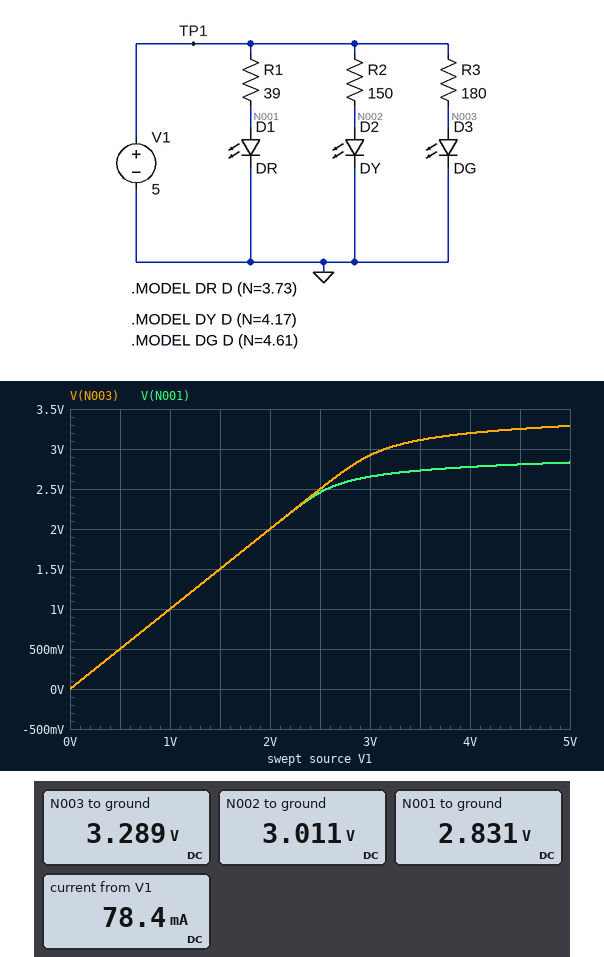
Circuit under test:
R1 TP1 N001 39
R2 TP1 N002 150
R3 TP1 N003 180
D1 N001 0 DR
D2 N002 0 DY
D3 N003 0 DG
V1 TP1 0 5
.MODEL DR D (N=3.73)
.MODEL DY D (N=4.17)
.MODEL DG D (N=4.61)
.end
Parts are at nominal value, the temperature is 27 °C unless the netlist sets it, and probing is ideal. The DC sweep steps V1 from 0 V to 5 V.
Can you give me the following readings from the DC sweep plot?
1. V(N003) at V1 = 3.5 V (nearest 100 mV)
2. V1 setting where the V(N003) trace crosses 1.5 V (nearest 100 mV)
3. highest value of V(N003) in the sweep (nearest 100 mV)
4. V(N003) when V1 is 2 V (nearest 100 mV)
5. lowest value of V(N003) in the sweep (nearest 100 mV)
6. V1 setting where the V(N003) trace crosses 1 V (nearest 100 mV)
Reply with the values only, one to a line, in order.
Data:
3.1 V
1.5 V
3.3 V
2.0 V
0 V
1.0 V
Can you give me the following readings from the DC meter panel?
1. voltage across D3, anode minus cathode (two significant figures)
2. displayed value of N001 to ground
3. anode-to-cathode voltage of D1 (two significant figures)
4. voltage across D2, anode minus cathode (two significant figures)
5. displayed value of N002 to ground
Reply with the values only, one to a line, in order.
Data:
3.3 V
2.831 V
2.8 V
3.0 V
3.011 V
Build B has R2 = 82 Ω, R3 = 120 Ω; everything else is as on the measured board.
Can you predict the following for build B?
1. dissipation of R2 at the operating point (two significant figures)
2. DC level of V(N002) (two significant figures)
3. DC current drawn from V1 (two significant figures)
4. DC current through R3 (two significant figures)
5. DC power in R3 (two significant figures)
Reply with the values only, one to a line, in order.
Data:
45 mW
3.1 V
93 mA
14 mA
23 mW
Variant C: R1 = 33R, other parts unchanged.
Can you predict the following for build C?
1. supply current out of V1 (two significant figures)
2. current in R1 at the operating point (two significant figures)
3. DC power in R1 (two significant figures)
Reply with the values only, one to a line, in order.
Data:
88 mA
65 mA
140 mW
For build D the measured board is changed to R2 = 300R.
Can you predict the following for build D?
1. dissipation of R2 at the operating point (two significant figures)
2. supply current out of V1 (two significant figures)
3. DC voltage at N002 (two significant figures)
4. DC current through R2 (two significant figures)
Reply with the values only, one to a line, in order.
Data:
14 mW
72 mA
2.9 V
6.9 mA
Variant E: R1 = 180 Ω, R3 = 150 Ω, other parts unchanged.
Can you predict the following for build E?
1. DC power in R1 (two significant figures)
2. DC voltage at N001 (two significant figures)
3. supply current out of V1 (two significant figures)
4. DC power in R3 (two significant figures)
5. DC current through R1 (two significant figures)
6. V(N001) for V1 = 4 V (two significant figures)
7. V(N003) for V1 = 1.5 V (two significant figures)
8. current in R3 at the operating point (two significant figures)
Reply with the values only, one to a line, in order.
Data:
30 mW
2.7 V
37 mA
19 mW
13 mA
2.6 V
1.5 V
11 mA
